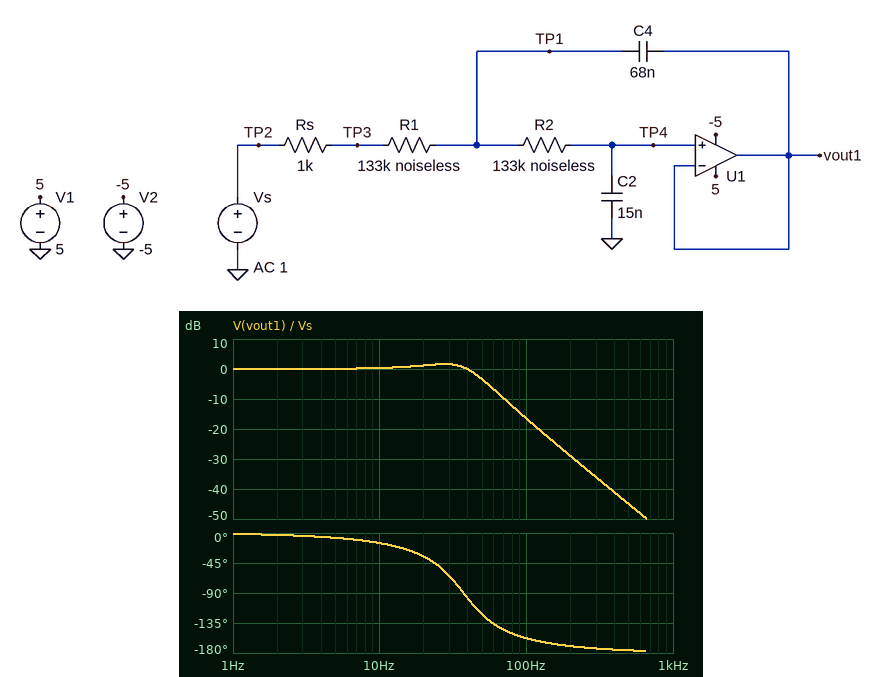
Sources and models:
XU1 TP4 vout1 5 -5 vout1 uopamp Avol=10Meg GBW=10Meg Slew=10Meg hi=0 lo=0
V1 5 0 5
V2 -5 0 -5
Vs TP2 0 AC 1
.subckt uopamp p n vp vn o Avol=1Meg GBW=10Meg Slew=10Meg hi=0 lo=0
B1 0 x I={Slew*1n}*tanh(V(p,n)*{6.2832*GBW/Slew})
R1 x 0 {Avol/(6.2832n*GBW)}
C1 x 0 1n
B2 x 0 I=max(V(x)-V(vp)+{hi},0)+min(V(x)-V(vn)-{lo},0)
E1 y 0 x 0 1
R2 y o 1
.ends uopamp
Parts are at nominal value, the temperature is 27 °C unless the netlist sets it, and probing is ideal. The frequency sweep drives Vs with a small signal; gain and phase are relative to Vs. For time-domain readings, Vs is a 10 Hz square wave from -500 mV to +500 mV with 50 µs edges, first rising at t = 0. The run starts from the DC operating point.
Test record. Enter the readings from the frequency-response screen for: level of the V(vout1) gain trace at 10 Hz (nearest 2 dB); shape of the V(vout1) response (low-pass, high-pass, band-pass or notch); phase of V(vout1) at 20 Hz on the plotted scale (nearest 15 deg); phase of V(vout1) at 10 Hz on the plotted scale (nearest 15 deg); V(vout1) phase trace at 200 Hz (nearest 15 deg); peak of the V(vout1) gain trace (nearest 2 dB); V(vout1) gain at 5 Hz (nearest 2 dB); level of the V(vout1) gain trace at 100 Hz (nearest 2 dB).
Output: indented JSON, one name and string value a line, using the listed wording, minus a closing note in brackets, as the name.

{
  "level of the V(vout1) gain trace at 10 Hz": "0 dB",
  "shape of the V(vout1) response": "low-pass",
  "phase of V(vout1) at 20 Hz on the plotted scale": "-30 deg",
  "phase of V(vout1) at 10 Hz on the plotted scale": "-15 deg",
  "V(vout1) phase trace at 200 Hz": "-165 deg",
  "peak of the V(vout1) gain trace": "2 dB",
  "V(vout1) gain at 5 Hz": "0 dB",
  "level of the V(vout1) gain trace at 100 Hz": "-16 dB"
}
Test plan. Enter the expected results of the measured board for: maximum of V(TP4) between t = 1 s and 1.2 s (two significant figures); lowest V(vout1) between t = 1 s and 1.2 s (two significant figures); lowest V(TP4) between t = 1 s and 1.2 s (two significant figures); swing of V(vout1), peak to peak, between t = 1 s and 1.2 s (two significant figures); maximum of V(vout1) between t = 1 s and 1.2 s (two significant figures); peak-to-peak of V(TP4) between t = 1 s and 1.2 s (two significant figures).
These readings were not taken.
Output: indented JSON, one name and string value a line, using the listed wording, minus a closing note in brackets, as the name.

{
  "maximum of V(TP4) between t = 1 s and 1.2 s": "690 mV",
  "lowest V(vout1) between t = 1 s and 1.2 s": "-690 mV",
  "lowest V(TP4) between t = 1 s and 1.2 s": "-690 mV",
  "swing of V(vout1), peak to peak, between t = 1 s and 1.2 s": "1.4 V",
  "maximum of V(vout1) between t = 1 s and 1.2 s": "690 mV",
  "peak-to-peak of V(TP4) between t = 1 s and 1.2 s": "1.4 V"
}
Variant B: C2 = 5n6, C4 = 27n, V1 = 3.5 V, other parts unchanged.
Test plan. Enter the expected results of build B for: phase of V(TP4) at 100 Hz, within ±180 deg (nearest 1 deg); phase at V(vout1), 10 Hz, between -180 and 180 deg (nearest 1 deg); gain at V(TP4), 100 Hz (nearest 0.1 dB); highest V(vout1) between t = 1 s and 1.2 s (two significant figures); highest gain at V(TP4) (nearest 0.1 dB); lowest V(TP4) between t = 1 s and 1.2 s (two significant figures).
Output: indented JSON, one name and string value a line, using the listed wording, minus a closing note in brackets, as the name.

{
  "phase of V(TP4) at 100 Hz, within ±180 deg": "-94 deg",
  "phase at V(vout1), 10 Hz, between -180 and 180 deg": "-5 deg",
  "gain at V(TP4), 100 Hz": "0.5 dB",
  "highest V(vout1) between t = 1 s and 1.2 s": "700 mV",
  "highest gain at V(TP4)": "1.8 dB",
  "lowest V(TP4) between t = 1 s and 1.2 s": "-700 mV"
}
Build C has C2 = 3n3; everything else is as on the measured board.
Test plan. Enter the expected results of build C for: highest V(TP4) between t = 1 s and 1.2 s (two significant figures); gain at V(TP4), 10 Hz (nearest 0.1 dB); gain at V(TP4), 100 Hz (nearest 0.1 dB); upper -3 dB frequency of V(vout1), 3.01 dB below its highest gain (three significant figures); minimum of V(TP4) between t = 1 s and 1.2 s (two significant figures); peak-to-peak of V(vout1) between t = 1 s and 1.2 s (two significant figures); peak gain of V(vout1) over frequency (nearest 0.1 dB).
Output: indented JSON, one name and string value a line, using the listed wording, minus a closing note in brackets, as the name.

{
  "highest V(TP4) between t = 1 s and 1.2 s": "990 mV",
  "gain at V(TP4), 10 Hz": "0.1 dB",
  "gain at V(TP4), 100 Hz": "1.9 dB",
  "upper -3 dB frequency of V(vout1), 3.01 dB below its highest gain": "91.9 Hz",
  "minimum of V(TP4) between t = 1 s and 1.2 s": "-990 mV",
  "peak-to-peak of V(vout1) between t = 1 s and 1.2 s": "2.0 V",
  "peak gain of V(vout1) over frequency": "7.3 dB"
}
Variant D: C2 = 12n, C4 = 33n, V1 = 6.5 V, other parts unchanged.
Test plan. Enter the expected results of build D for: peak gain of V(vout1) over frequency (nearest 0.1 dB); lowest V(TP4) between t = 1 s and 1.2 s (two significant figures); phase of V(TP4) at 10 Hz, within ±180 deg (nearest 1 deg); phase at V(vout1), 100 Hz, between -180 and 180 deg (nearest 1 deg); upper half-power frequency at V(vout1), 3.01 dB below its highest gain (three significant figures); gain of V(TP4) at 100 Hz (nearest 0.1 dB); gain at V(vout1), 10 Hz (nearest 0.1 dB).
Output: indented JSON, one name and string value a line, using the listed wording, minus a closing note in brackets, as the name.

{
  "peak gain of V(vout1) over frequency": "0.3 dB",
  "lowest V(TP4) between t = 1 s and 1.2 s": "-590 mV",
  "phase of V(TP4) at 10 Hz, within ±180 deg": "-12 deg",
  "phase at V(vout1), 100 Hz, between -180 and 180 deg": "-132 deg",
  "upper half-power frequency at V(vout1), 3.01 dB below its highest gain": "66.6 Hz",
  "gain of V(TP4) at 100 Hz": "-8.6 dB",
  "gain at V(vout1), 10 Hz": "0.1 dB"
}
